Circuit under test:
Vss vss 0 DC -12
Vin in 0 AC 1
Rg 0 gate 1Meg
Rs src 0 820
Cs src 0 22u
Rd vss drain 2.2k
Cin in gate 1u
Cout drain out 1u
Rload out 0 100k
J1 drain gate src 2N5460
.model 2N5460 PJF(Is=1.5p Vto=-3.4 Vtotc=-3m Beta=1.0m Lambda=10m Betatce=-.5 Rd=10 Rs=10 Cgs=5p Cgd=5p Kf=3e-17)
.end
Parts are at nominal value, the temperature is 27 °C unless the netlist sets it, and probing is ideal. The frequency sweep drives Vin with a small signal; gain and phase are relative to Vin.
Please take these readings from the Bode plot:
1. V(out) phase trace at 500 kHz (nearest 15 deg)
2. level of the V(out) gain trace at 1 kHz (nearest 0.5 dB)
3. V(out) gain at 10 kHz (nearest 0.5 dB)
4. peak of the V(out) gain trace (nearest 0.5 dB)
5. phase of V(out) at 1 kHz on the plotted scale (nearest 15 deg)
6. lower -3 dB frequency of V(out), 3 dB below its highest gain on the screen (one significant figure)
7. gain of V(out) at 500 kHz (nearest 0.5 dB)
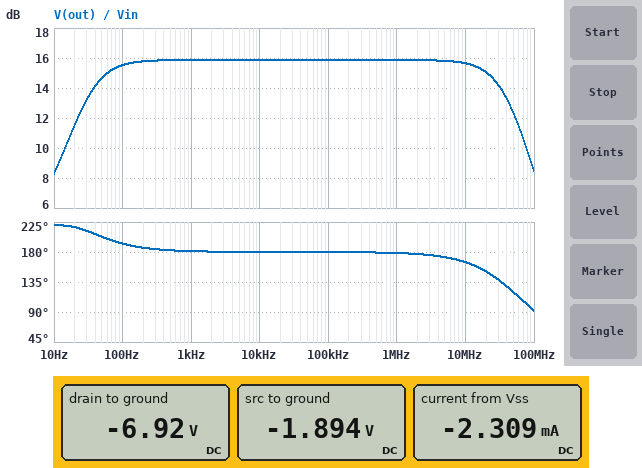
180 deg
16.0 dB
16.0 dB
16.0 dB
180 deg
30 Hz
16.0 dB
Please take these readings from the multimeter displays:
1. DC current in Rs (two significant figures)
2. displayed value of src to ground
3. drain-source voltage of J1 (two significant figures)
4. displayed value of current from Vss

2.3 mA
-1.894 V
-5.0 V
-2.309 mA
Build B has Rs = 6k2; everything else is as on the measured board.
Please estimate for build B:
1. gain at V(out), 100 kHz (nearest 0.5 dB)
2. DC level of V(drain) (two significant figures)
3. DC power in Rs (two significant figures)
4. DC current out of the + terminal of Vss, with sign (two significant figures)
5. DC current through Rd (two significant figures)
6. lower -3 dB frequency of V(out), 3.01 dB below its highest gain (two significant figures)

9.5 dB
-11 V
1.2 mW
-440 µA
440 µA
11 Hz
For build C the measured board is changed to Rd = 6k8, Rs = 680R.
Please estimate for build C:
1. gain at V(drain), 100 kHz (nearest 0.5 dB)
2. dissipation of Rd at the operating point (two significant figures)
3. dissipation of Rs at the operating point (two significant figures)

-15.0 dB
16 mW
1.6 mW
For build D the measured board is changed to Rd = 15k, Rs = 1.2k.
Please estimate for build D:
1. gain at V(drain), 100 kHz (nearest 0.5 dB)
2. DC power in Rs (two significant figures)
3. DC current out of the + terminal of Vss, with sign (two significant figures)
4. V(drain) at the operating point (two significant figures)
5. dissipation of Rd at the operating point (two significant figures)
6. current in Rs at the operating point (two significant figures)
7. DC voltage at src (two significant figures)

-24.0 dB
640 µW
-730 µA
-1.0 V
8.0 mW
730 µA
-880 mV
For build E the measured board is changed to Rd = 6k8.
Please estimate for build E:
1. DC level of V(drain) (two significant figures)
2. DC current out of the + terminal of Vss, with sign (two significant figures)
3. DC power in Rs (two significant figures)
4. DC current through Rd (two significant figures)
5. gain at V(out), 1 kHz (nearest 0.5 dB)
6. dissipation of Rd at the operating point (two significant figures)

-1.7 V
-1.5 mA
1.9 mW
1.5 mA
-13.5 dB
16 mW
